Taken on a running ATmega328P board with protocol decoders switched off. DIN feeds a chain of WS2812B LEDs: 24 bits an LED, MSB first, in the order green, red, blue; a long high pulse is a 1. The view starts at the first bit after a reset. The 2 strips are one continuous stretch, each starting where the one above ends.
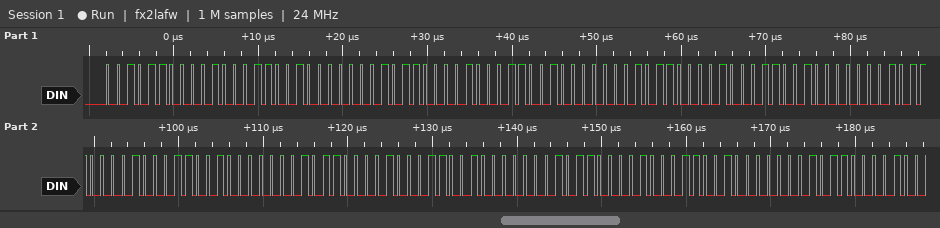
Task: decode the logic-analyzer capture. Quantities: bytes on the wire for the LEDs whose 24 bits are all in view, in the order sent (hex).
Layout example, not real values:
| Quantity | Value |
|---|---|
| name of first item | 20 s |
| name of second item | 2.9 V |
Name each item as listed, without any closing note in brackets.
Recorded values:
| Quantity | Value |
|---|---|
| bytes on the wire for the LEDs whose 24 bits are all in view, in the order sent | 2C 23 20 2C 23 20 2C 23 20 2C 23 20 2C 23 20 2C 23 20 |
